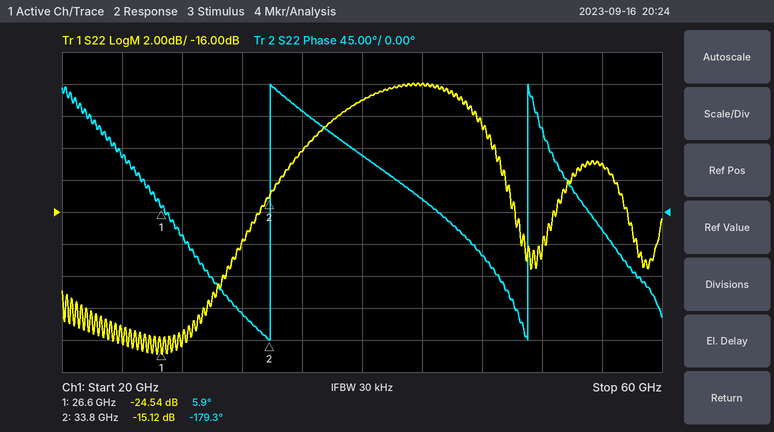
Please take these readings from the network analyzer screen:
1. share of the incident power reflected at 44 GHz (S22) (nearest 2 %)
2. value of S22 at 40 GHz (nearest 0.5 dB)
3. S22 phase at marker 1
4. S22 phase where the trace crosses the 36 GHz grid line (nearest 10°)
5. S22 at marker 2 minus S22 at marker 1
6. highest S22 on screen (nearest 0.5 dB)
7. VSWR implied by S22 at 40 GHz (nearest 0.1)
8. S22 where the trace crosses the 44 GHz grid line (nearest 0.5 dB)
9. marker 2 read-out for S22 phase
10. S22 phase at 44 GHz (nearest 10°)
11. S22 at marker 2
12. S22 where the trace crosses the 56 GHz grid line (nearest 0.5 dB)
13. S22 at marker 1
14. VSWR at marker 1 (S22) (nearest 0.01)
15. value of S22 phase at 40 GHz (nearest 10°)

16 %
-9.0 dB
5.9°
140°
9.42 dB
-8.0 dB
2.1
-8.0 dB
-179.3°
20°
-15.12 dB
-13.0 dB
-24.54 dB
1.13
80°
